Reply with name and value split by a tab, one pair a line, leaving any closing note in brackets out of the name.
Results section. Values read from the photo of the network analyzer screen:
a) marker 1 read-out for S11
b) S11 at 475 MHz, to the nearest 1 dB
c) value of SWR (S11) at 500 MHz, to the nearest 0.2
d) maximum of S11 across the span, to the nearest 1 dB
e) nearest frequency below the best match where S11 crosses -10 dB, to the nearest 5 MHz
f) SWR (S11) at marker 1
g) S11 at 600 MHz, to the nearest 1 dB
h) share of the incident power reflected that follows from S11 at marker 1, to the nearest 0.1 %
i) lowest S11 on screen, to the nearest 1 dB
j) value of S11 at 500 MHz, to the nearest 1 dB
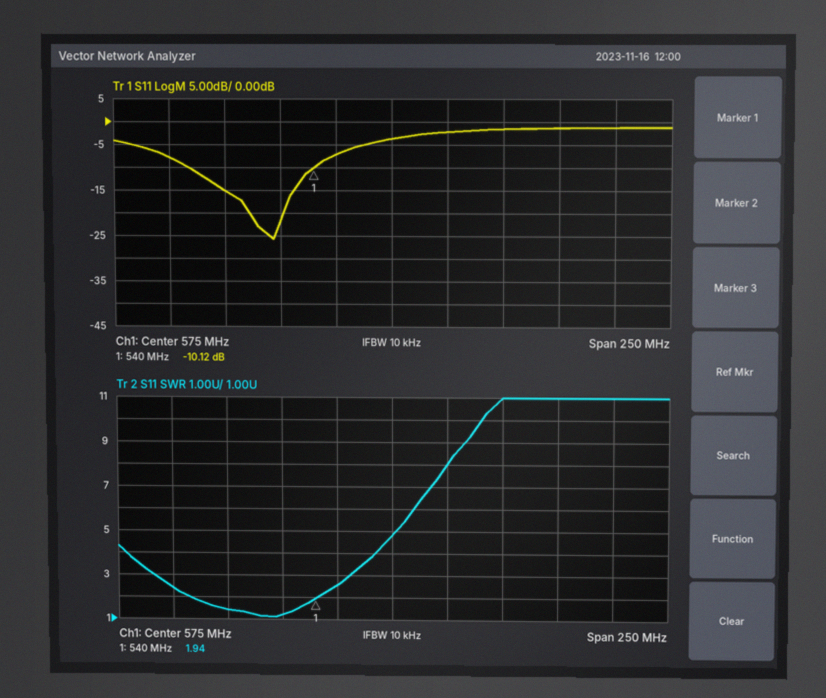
marker 1 read-out for S11	-10.12 dB
S11 at 475 MHz, to the nearest 1 dB	-8 dB
value of SWR (S11) at 500 MHz, to the nearest 0.2	1.4
maximum of S11 across the span, to the nearest 1 dB	-1 dB
nearest frequency below the best match where S11 crosses -10 dB, to the nearest 5 MHz	485 MHz
SWR (S11) at marker 1	1.94
S11 at 600 MHz, to the nearest 1 dB	-2 dB
share of the incident power reflected that follows from S11 at marker 1, to the nearest 0.1 %	9.7 %
lowest S11 on screen, to the nearest 1 dB	-26 dB
value of S11 at 500 MHz, to the nearest 1 dB	-15 dB
